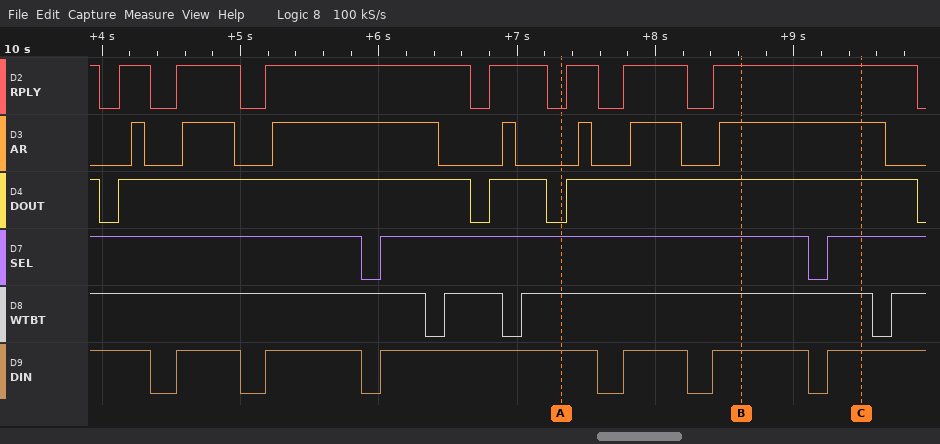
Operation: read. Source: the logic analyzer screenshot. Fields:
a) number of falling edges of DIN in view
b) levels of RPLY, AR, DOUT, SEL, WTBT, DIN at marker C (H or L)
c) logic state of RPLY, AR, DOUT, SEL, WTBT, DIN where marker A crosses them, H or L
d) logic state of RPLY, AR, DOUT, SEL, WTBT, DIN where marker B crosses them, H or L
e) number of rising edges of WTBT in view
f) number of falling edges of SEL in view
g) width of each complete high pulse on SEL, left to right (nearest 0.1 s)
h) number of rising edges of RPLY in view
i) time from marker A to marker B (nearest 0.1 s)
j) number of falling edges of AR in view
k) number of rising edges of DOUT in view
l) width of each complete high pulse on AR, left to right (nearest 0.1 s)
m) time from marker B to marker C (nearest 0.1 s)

6
RPLY=H, AR=H, DOUT=H, SEL=H, WTBT=H, DIN=H
RPLY=L, AR=L, DOUT=L, SEL=H, WTBT=H, DIN=H
RPLY=H, AR=H, DOUT=H, SEL=H, WTBT=H, DIN=H
3
2
3.1 s
7
1.3 s
7
3
0.1 s, 0.4 s, 1.2 s, 0.1 s, 0.1 s, 0.4 s, 1.2 s
0.9 s
